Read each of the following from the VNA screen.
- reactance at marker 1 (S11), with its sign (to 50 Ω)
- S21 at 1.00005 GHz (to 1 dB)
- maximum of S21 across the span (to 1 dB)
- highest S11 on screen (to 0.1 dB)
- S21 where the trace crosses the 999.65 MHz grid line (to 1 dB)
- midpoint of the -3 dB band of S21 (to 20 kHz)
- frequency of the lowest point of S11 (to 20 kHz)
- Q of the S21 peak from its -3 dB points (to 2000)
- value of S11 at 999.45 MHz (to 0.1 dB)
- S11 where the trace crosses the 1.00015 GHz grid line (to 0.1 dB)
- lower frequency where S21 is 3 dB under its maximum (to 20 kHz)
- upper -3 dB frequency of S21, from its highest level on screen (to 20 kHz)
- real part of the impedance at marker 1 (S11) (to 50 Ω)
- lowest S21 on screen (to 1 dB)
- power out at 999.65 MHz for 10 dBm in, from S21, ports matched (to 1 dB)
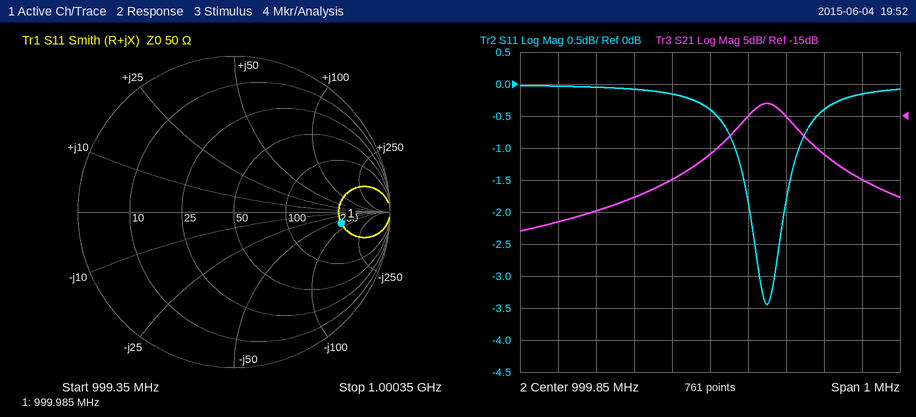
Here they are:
-50 Ω
-15 dB
-13 dB
0.0 dB
-28 dB
1.00000 GHz
1.00000 GHz
8000
0.0 dB
-0.4 dB
999.94 MHz
1.00006 GHz
250 Ω
-33 dB
-18 dBm
